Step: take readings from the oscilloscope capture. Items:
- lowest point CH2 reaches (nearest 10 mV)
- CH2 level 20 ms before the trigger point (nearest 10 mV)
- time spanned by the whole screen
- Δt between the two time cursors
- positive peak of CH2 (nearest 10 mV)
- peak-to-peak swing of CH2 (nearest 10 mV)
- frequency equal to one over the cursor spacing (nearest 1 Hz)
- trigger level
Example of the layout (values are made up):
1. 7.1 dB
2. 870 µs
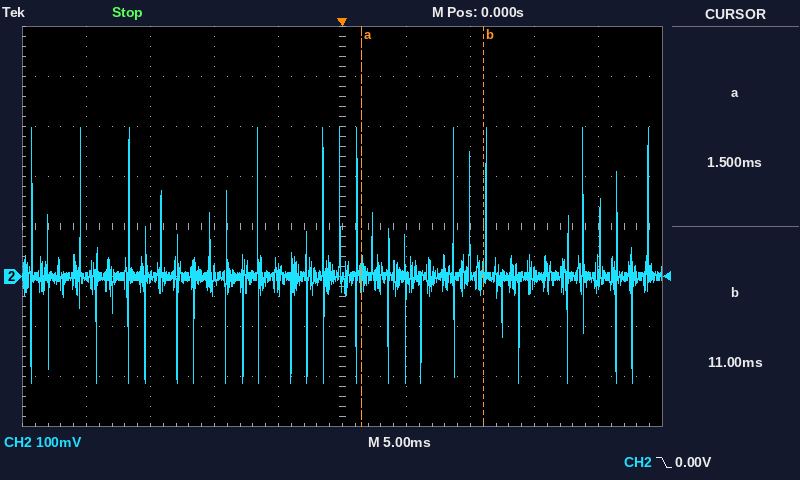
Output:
1. -210 mV
2. 0 mV
3. 50 ms
4. 9.5 ms
5. 300 mV
6. 510 mV
7. 105 Hz
8. 0.00 V
